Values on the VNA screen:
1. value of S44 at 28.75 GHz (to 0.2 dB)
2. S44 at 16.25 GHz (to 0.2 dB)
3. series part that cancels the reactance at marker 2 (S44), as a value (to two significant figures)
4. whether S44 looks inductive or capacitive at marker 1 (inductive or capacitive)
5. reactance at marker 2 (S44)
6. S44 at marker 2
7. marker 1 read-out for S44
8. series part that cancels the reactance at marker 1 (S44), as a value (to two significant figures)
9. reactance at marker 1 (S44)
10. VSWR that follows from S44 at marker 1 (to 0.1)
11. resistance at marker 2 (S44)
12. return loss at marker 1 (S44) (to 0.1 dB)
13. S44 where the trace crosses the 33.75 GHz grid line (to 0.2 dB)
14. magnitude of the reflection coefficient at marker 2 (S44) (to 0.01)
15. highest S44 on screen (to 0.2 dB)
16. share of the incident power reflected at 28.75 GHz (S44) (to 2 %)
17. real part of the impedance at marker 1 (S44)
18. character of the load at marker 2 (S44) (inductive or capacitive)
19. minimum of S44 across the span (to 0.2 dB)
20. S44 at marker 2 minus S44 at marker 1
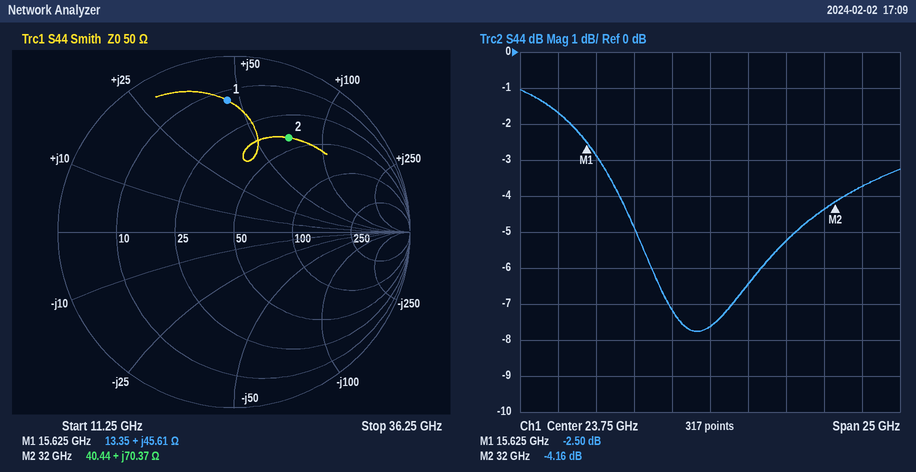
-5.2 dB
-2.8 dB
71 fF
inductive
+70.37 Ω
-4.16 dB
-2.50 dB
220 fF
+45.61 Ω
7.0
40.44 Ω
2.5 dB
-3.8 dB
0.62
-1.0 dB
30 %
13.35 Ω
inductive
-7.8 dB
-1.66 dB
